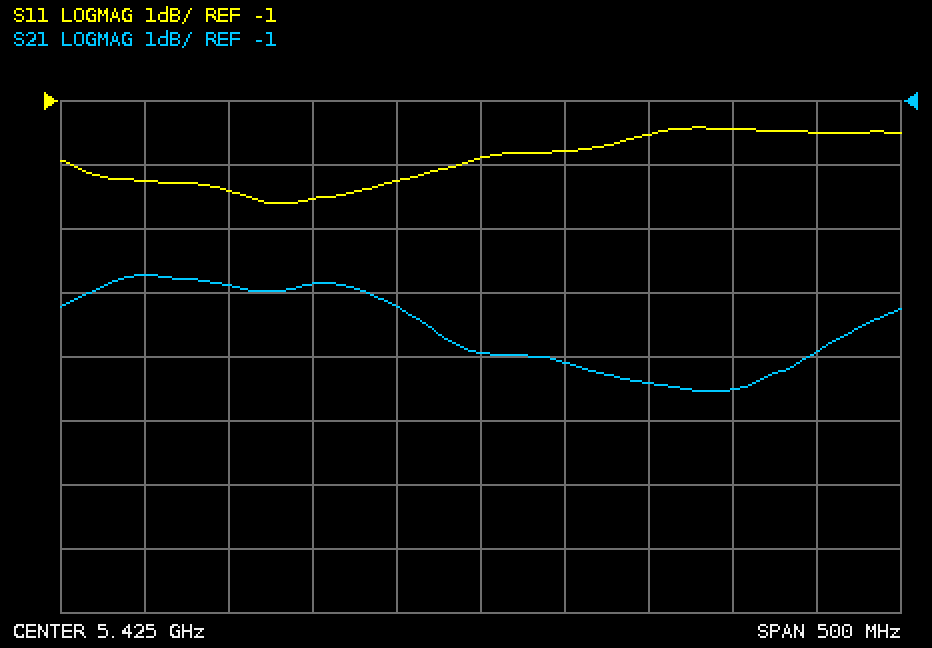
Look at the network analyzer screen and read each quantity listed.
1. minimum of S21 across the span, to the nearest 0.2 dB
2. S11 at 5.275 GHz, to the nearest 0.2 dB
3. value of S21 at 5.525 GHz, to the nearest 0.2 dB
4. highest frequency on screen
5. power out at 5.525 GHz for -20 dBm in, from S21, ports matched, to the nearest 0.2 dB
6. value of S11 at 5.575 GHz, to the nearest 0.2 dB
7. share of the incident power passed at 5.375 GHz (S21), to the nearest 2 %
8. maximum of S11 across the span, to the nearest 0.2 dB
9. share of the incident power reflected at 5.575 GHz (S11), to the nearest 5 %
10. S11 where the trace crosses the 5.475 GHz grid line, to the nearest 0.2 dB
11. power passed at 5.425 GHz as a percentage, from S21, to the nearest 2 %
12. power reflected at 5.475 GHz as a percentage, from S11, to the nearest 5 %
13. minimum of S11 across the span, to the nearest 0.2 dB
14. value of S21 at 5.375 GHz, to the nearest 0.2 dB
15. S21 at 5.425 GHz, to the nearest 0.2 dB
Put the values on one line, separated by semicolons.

-5.6 dB; -2.4 dB; -5.4 dB; 5.675 GHz; -25.4 dBm; -1.4 dB; 38 %; -1.4 dB; 70 %; -1.8 dB; 32 %; 65 %; -2.6 dB; -4.2 dB; -5.0 dB
